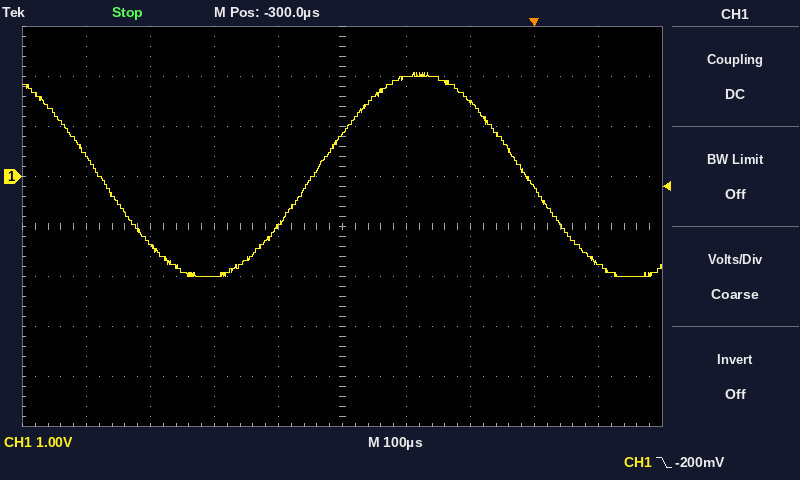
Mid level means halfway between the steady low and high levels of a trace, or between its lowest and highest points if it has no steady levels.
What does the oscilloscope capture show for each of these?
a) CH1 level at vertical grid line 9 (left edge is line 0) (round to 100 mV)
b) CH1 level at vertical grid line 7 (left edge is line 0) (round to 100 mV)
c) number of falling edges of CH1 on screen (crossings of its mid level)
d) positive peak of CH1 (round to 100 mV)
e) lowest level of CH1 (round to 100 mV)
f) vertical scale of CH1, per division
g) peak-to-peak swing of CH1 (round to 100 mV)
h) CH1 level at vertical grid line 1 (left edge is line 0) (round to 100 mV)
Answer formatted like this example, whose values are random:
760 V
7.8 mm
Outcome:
-1.7 V
1.5 V
2
2.1 V
-2.0 V
1 V
4.1 V
400 mV
